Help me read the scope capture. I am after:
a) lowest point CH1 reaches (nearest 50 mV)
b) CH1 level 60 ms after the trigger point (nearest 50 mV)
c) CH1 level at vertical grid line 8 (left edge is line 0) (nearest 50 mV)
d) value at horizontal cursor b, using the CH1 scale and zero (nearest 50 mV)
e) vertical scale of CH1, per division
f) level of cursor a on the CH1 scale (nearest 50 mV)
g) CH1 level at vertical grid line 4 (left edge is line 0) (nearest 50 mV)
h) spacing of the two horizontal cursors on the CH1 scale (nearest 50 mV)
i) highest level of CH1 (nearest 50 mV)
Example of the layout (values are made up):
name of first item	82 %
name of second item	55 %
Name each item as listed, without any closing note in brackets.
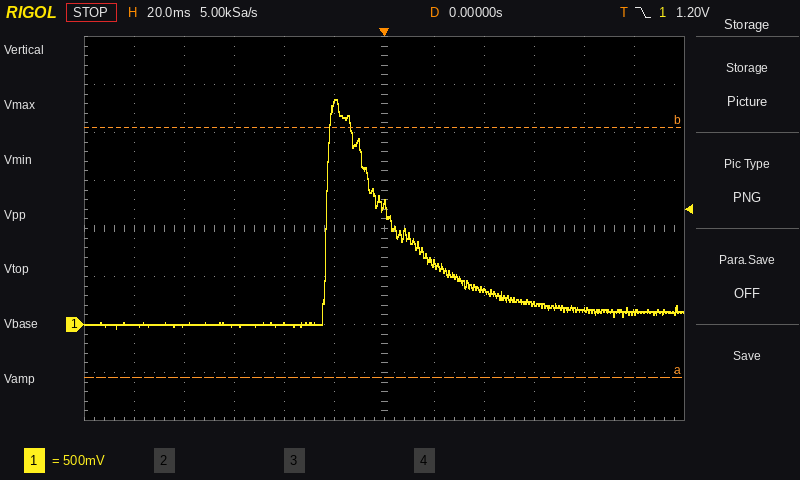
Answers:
lowest point CH1 reaches	-50 mV
CH1 level 60 ms after the trigger point	200 mV
CH1 level at vertical grid line 8 (left edge is line 0)	350 mV
value at horizontal cursor b, using the CH1 scale and zero	2.05 V
vertical scale of CH1, per division	500 mV
level of cursor a on the CH1 scale	-550 mV
CH1 level at vertical grid line 4 (left edge is line 0)	0 mV
spacing of the two horizontal cursors on the CH1 scale	2.60 V
highest level of CH1	2.35 V
